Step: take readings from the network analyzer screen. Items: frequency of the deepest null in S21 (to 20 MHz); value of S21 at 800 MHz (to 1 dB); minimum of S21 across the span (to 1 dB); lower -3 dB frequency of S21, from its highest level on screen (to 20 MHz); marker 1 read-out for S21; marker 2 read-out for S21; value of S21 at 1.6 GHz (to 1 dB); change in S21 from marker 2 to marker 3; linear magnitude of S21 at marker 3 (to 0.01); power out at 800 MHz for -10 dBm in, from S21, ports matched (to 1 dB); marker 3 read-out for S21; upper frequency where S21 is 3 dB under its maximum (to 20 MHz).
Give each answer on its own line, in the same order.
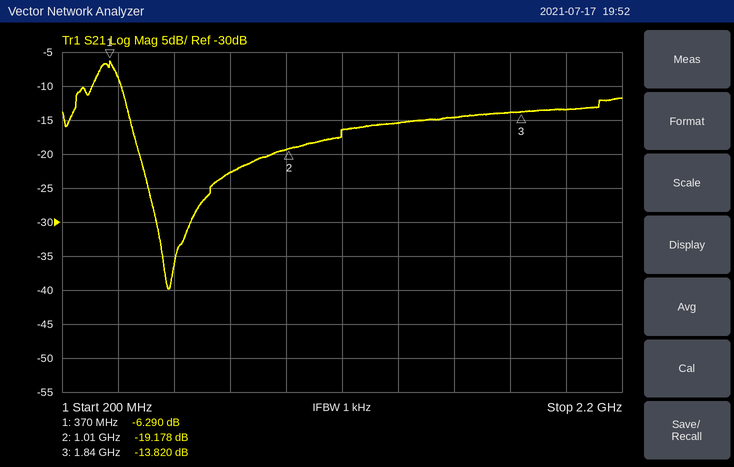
580 MHz
-23 dB
-40 dB
320 MHz
-6.290 dB
-19.178 dB
-15 dB
5.358 dB
0.20
-33 dBm
-13.820 dB
400 MHz
